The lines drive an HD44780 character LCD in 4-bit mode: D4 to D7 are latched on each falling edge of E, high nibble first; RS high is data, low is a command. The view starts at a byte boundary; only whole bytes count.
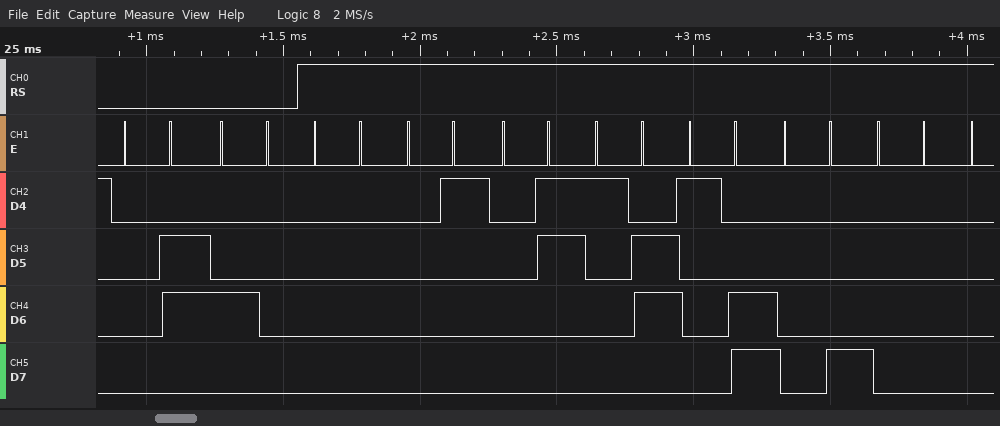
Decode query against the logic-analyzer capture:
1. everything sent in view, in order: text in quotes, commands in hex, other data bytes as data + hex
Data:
0x06 0x40 data 00 01 03 16 1C 08 00
